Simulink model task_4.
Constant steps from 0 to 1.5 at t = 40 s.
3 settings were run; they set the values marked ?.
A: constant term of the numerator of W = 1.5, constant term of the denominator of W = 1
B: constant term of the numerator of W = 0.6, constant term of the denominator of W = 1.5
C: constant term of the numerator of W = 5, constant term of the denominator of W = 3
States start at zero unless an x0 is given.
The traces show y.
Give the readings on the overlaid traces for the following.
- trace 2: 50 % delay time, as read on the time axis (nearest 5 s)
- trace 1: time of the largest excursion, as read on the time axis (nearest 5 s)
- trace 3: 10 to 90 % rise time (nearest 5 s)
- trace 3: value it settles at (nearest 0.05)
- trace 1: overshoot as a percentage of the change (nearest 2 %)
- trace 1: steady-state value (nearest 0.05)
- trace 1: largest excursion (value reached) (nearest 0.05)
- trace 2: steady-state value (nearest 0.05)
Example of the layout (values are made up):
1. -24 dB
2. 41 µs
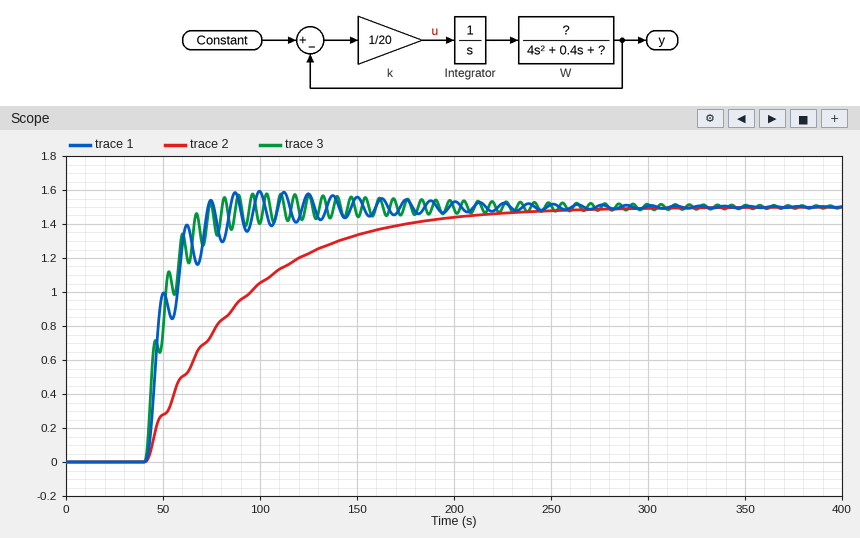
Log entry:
1. 75 s
2. 100 s
3. 25 s
4. 1.50
5. 6 %
6. 1.50
7. 1.60
8. 1.50
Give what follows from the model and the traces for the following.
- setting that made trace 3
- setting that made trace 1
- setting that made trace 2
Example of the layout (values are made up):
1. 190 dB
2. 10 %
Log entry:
1. C
2. A
3. B
